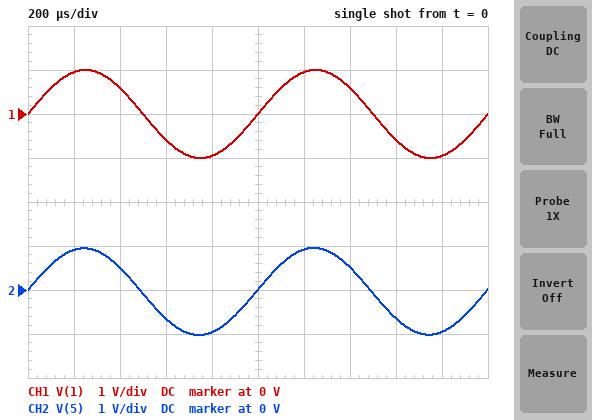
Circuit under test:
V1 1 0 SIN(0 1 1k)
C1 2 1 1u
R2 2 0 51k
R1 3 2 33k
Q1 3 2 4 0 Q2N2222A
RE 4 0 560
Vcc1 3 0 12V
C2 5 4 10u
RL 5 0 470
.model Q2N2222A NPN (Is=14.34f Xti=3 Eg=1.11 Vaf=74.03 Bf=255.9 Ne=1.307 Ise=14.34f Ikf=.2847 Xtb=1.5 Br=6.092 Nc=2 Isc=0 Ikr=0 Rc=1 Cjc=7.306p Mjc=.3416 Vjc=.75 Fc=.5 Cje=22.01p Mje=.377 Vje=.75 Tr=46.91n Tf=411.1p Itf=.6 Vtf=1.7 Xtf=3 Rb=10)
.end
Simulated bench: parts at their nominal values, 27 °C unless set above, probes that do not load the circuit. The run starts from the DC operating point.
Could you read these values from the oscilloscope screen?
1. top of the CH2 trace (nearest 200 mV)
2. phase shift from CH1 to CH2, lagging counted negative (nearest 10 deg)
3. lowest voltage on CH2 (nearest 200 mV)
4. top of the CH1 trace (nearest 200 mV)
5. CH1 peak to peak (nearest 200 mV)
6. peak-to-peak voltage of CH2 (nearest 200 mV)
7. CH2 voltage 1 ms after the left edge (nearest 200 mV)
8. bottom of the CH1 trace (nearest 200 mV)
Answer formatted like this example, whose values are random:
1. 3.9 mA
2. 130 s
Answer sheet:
1. 1.0 V
2. 0 deg
3. -1.0 V
4. 1.0 V
5. 2.0 V
6. 2.0 V
7. 0 V
8. -1.0 V
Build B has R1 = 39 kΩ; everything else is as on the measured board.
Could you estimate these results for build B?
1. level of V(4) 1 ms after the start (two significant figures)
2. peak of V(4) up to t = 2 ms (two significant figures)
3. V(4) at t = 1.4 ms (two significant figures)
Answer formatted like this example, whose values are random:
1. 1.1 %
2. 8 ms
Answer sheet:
1. 5.0 V
2. 6.0 V
3. 5.6 V
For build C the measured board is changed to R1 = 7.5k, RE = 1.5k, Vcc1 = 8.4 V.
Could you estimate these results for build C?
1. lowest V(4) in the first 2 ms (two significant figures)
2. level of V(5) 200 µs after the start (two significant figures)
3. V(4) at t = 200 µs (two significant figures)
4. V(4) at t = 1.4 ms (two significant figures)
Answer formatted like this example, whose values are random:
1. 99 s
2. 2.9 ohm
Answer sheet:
1. 5.5 V
2. 900 mV
3. 7.4 V
4. 7.0 V
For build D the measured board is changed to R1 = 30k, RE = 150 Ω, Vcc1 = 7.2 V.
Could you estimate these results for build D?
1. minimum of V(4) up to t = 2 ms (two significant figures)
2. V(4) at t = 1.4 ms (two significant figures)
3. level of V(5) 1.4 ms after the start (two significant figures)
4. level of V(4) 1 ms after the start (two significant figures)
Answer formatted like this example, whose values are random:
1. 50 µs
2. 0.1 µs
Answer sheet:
1. 1.3 V
2. 2.8 V
3. 500 mV
4. 2.3 V
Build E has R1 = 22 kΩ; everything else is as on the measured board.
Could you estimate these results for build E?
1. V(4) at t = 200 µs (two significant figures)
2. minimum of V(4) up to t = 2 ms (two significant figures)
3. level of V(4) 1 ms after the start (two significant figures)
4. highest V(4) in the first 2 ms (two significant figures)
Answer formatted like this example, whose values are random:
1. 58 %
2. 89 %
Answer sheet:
1. 7.6 V
2. 5.7 V
3. 6.7 V
4. 7.7 V
